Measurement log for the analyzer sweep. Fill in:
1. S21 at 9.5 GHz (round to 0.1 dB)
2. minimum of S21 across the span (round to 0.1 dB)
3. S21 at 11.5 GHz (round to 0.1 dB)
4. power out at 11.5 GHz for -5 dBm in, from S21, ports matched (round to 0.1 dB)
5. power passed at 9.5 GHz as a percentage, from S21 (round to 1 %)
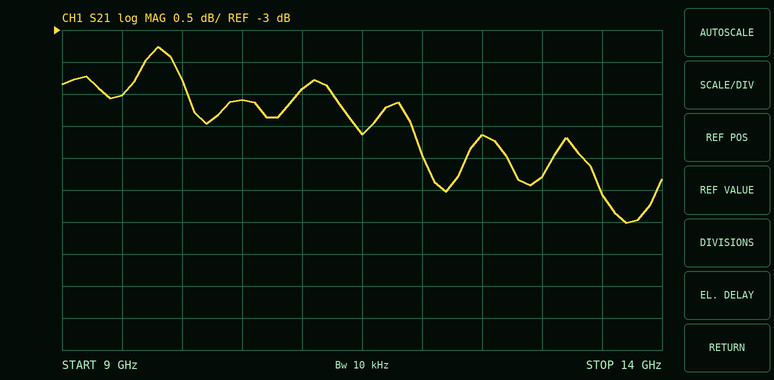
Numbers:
-4.0 dB
-6.0 dB
-4.6 dB
-9.6 dBm
40 %
